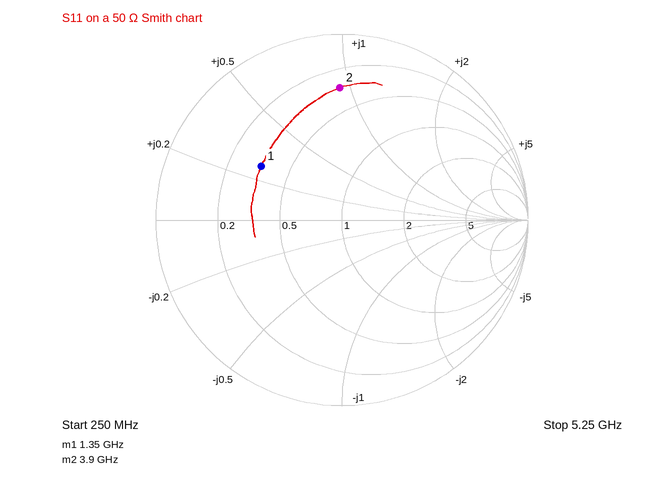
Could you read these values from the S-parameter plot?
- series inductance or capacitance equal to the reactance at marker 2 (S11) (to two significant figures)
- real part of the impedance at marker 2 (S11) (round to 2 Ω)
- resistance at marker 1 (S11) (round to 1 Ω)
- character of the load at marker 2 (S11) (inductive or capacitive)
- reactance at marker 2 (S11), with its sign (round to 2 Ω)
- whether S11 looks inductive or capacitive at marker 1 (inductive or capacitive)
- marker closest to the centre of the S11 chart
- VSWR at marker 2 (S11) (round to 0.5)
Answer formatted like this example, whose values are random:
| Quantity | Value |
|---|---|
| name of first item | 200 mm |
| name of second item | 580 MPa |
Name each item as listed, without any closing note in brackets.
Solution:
| Quantity | Value |
|---|---|
| series inductance or capacitance equal to the reactance at marker 2 (S11) | 1.9 nH |
| real part of the impedance at marker 2 (S11) | 16 Ω |
| resistance at marker 1 (S11) | 17 Ω |
| character of the load at marker 2 (S11) | inductive |
| reactance at marker 2 (S11), with its sign | +46 Ω |
| whether S11 looks inductive or capacitive at marker 1 | inductive |
| marker closest to the centre of the S11 chart | marker 1 |
| VSWR at marker 2 (S11) | 6.0 |
